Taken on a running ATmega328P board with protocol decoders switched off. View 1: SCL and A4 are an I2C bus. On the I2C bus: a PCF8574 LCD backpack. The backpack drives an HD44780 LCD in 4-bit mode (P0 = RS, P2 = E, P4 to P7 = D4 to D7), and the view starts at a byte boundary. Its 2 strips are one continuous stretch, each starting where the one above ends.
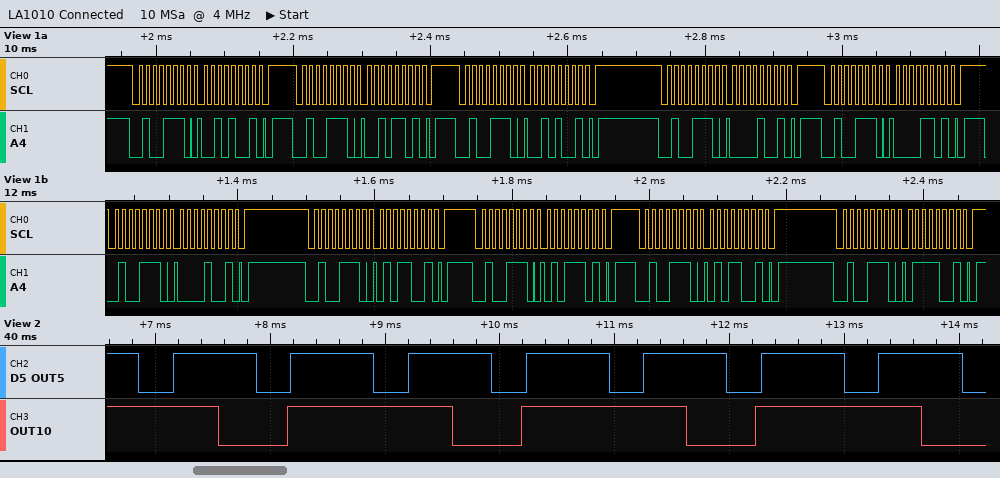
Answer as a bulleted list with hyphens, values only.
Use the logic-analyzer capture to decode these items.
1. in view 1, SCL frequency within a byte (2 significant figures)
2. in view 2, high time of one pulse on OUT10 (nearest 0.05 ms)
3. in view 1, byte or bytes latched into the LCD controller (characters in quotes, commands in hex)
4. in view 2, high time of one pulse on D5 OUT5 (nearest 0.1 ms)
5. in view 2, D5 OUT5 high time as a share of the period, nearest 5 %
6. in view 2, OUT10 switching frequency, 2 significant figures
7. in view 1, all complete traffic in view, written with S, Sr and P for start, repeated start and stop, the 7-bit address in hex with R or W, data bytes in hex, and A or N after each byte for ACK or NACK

- 100 kHz
- 1.45 ms
- ' '
- 0.7 ms
- 70 %
- 490 Hz
- S 27W A 29 A P S 27W A 2D A P S 27W A 29 A P S 27W A 09 A P S 27W A 0D A P S 27W A 09 A P S 27W A 59 A P S 27W A 5D A P S 27W A 59 A P S 27W A 79 A P
